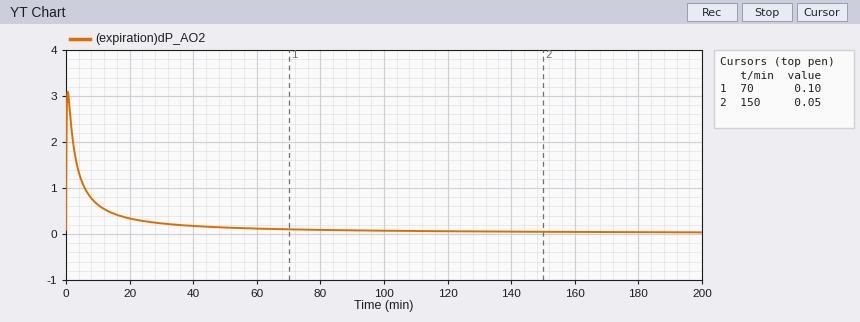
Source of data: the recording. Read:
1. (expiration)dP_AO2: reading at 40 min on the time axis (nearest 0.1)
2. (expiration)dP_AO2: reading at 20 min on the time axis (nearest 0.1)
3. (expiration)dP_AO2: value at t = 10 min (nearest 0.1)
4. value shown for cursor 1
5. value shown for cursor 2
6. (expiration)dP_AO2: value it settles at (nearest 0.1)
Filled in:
0.2
0.3
0.6
0.10
0.05
0.0
